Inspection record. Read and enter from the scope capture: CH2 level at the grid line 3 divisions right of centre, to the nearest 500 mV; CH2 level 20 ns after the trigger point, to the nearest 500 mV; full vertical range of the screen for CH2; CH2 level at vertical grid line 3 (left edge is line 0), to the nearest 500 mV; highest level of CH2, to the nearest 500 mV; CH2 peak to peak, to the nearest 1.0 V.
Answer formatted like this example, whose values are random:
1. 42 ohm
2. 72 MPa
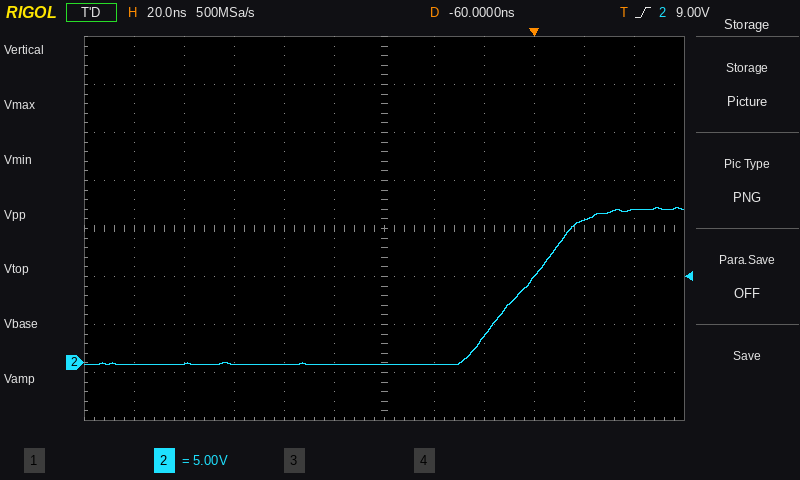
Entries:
1. 9.0 V
2. 15.0 V
3. 40 V
4. 0.0 V
5. 16.0 V
6. 16.0 V
